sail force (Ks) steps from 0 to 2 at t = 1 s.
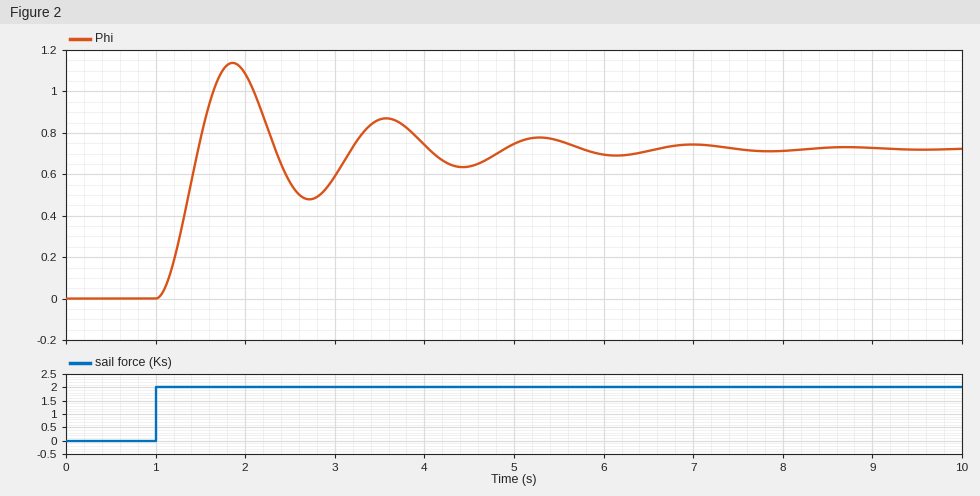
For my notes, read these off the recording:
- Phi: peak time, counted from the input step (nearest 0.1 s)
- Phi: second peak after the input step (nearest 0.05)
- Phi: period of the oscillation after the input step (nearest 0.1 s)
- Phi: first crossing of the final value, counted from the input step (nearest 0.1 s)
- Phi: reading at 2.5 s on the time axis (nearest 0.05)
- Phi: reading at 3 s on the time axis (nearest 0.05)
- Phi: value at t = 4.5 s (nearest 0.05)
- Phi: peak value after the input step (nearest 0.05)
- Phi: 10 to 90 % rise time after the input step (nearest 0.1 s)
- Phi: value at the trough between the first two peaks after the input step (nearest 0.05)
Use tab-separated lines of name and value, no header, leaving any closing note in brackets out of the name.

Phi: peak time, counted from the input step	0.9 s
Phi: second peak after the input step	0.85
Phi: period of the oscillation after the input step	1.7 s
Phi: first crossing of the final value, counted from the input step	0.5 s
Phi: reading at 2.5 s on the time axis	0.55
Phi: reading at 3 s on the time axis	0.60
Phi: value at t = 4.5 s	0.65
Phi: peak value after the input step	1.15
Phi: 10 to 90 % rise time after the input step	0.3 s
Phi: value at the trough between the first two peaks after the input step	0.50
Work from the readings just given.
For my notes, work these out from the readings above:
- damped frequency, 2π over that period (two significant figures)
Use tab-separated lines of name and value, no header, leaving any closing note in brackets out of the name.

damped frequency, 2π over that period	3.7 rad/s
